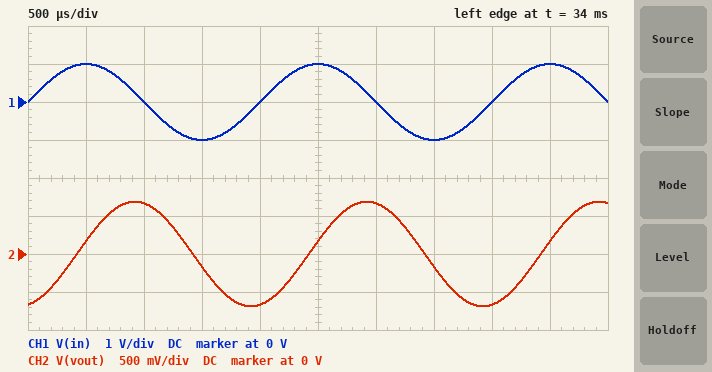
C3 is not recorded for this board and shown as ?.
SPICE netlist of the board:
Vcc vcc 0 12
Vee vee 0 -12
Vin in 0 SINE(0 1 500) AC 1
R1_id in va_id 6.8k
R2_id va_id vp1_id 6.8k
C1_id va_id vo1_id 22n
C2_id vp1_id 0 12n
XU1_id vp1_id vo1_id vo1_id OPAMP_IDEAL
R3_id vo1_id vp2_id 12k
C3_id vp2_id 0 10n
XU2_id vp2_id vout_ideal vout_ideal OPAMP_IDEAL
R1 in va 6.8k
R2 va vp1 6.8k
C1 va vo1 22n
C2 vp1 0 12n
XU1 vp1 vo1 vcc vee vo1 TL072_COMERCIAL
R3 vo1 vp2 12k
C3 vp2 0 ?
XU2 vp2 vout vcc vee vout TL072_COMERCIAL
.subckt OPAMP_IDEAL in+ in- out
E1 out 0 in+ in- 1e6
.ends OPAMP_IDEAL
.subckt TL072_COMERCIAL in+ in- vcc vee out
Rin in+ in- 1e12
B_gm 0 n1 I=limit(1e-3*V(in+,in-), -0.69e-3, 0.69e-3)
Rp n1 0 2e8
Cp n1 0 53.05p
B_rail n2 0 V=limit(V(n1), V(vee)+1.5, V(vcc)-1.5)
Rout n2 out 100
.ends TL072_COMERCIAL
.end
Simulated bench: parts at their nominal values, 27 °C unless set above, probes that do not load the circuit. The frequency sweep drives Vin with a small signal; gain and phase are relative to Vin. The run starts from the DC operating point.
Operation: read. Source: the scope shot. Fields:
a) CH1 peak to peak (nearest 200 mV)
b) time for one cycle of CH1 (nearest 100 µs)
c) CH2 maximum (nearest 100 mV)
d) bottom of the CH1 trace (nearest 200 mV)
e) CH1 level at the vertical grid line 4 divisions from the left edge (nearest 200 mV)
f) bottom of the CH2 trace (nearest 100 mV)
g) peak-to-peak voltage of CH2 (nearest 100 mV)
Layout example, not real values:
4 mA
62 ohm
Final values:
2.0 V
2.0 ms
700 mV
-1.0 V
0 V
-700 mV
1.4 V
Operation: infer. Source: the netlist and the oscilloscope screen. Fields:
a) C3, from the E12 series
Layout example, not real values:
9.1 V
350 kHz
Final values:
27 nF
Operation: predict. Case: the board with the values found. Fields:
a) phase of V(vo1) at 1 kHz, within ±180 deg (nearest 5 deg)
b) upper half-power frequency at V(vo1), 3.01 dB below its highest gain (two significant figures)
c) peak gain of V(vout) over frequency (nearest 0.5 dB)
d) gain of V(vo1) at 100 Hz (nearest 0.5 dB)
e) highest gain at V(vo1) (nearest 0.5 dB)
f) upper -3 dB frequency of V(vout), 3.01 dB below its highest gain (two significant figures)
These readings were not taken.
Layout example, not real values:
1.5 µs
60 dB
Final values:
-65 deg
1.4 kHz
0 dB
0 dB
0 dB
480 Hz
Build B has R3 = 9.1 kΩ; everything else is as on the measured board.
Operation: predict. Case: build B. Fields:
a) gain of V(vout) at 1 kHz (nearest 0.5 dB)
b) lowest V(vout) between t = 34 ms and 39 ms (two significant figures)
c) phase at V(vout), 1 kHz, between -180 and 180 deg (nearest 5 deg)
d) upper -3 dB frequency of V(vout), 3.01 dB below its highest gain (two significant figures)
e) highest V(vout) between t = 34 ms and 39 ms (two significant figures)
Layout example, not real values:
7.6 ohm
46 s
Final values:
-6.5 dB
-780 mV
-120 deg
610 Hz
780 mV
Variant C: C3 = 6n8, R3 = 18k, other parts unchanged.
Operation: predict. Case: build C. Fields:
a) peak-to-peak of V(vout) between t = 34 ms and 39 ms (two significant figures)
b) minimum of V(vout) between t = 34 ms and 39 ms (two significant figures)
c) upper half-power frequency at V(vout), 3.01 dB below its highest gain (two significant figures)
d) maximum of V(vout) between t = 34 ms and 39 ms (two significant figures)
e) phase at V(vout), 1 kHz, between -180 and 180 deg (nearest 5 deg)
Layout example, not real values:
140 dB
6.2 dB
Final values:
1.8 V
-920 mV
970 Hz
920 mV
-100 deg
